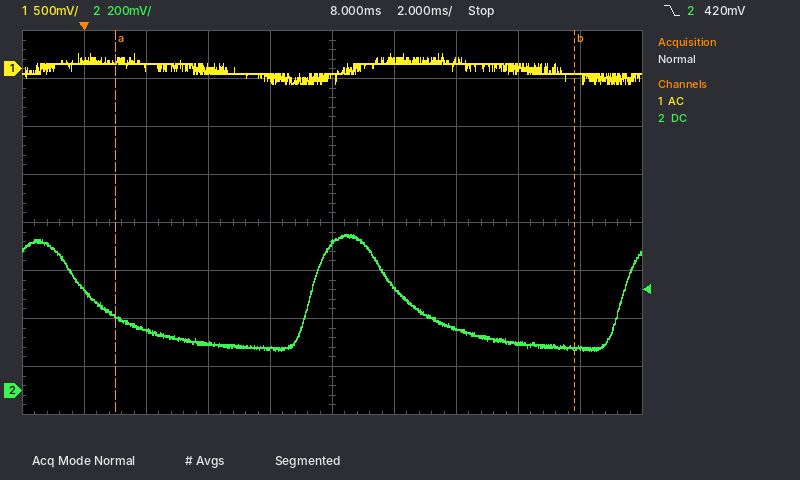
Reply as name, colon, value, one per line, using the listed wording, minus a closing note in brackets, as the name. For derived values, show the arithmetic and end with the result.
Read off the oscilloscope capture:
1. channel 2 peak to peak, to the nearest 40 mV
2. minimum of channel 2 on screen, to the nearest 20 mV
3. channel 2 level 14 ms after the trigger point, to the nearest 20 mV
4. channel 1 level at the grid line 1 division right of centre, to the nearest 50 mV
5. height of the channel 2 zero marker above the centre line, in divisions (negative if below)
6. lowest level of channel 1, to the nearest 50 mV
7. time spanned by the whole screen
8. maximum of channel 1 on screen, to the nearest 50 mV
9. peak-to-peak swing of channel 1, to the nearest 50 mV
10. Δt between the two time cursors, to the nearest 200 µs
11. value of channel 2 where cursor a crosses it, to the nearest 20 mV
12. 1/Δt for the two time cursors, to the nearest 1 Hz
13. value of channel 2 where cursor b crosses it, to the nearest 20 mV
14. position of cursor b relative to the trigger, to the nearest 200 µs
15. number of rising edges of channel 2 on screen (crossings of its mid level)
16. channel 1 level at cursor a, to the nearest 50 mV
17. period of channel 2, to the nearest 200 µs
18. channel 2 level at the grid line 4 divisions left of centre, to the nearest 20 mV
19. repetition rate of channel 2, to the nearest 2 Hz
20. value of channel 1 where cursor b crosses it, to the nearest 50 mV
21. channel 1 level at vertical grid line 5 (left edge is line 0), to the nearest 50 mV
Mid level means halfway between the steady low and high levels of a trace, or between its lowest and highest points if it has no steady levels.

channel 2 peak to peak, to the nearest 40 mV: 480 mV
minimum of channel 2 on screen, to the nearest 20 mV: 160 mV
channel 2 level 14 ms after the trigger point, to the nearest 20 mV: 200 mV
channel 1 level at the grid line 1 division right of centre, to the nearest 50 mV: 100 mV
height of the channel 2 zero marker above the centre line, in divisions: -3.5 div
lowest level of channel 1, to the nearest 50 mV: -150 mV
time spanned by the whole screen: 20 ms
maximum of channel 1 on screen, to the nearest 50 mV: 150 mV
peak-to-peak swing of channel 1, to the nearest 50 mV: 150 mV − (-150 mV) = 300 mV
Δt between the two time cursors, to the nearest 200 µs: 14.8 ms
value of channel 2 where cursor a crosses it, to the nearest 20 mV: 300 mV
1/Δt for the two time cursors, to the nearest 1 Hz: 1 / 14.8 ms ≈ 68 Hz
value of channel 2 where cursor b crosses it, to the nearest 20 mV: 180 mV
position of cursor b relative to the trigger, to the nearest 200 µs: +15.8 ms
number of rising edges of channel 2 on screen: 2
channel 1 level at cursor a, to the nearest 50 mV: 100 mV
period of channel 2, to the nearest 200 µs: 10.0 ms
channel 2 level at the grid line 4 divisions left of centre, to the nearest 20 mV: 420 mV
repetition rate of channel 2, to the nearest 2 Hz: 1 / 10.0 ms ≈ 100 Hz
value of channel 1 where cursor b crosses it, to the nearest 50 mV: -50 mV
channel 1 level at vertical grid line 5 (left edge is line 0), to the nearest 50 mV: -50 mV
